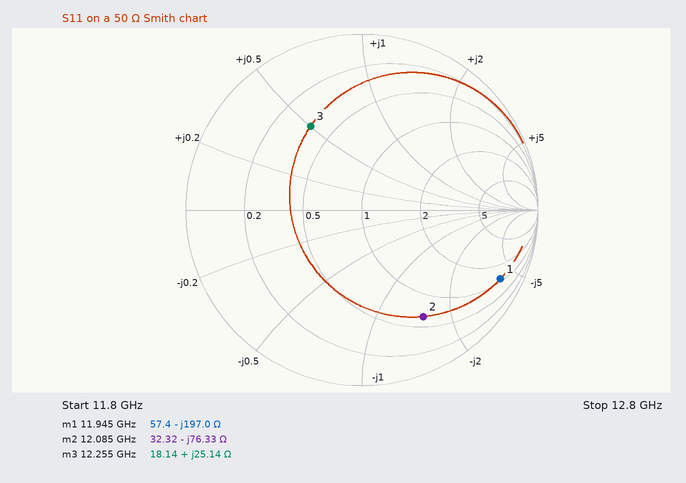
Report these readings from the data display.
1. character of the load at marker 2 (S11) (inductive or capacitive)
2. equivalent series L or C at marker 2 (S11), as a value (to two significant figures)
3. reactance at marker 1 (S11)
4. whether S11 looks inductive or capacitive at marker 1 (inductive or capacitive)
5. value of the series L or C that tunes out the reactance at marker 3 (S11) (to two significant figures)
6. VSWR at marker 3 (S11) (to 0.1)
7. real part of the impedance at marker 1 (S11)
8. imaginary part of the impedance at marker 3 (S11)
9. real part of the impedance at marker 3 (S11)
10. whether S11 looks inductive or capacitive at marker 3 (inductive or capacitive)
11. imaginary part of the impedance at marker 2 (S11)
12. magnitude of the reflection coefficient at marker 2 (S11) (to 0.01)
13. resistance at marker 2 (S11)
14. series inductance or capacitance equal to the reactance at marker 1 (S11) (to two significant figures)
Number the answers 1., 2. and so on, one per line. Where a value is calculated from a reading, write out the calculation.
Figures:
1. capacitive
2. C = 1/(2π × 12.085 GHz × 76.33 Ω) ≈ 173 fF, so 170 fF to two significant figures
3. -197.0 Ω
4. capacitive
5. C = 1/(2π × 12.255 GHz × 25.14 Ω) ≈ 517 fF, so 520 fF to two significant figures
6. 3.5
7. 57.4 Ω
8. +25.14 Ω
9. 18.14 Ω
10. inductive
11. -76.33 Ω
12. 0.70
13. 32.32 Ω
14. C = 1/(2π × 11.945 GHz × 197 Ω) ≈ 68 fF
